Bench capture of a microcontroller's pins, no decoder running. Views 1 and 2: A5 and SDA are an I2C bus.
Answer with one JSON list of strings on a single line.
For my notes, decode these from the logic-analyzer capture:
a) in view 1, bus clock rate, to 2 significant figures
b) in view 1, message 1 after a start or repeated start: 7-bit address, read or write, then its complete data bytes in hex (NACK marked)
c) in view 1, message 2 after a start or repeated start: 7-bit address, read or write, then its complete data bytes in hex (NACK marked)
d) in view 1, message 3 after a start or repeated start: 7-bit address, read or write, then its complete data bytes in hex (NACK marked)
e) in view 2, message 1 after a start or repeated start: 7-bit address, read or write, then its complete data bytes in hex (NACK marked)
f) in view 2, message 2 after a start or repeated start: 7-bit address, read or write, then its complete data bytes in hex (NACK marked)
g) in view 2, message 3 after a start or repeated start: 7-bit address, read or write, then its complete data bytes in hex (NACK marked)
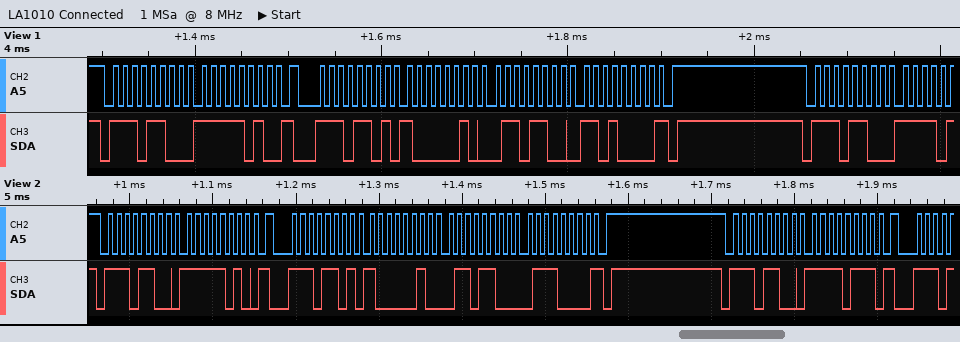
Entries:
["100 kHz", "0x76 write: FA", "0x76 read: 82 6C D0 NACK", "0x76 write", "0x76 write: FA", "0x76 read: 82 6C 70 NACK", "0x76 write: F7"]
